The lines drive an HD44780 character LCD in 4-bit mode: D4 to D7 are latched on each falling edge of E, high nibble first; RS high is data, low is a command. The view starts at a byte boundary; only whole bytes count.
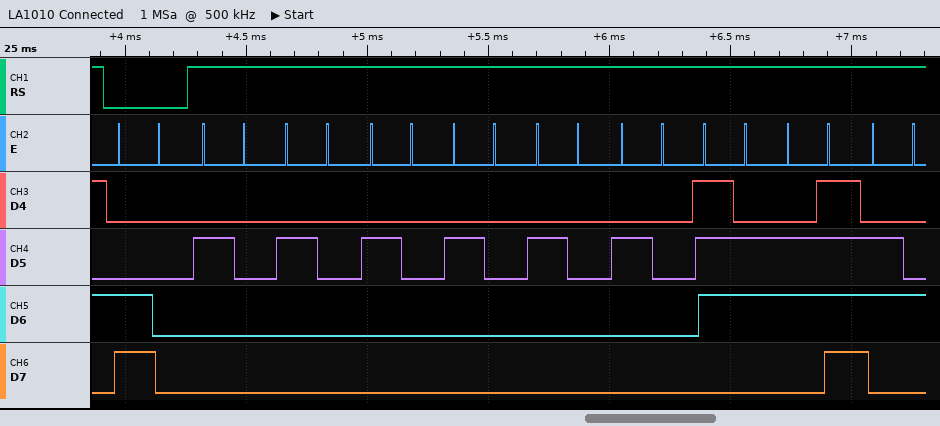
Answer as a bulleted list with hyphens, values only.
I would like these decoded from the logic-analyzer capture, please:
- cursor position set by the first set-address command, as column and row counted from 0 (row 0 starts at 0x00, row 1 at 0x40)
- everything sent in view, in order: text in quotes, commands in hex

- column 0, row 1
- 0xC0 "      vod"
